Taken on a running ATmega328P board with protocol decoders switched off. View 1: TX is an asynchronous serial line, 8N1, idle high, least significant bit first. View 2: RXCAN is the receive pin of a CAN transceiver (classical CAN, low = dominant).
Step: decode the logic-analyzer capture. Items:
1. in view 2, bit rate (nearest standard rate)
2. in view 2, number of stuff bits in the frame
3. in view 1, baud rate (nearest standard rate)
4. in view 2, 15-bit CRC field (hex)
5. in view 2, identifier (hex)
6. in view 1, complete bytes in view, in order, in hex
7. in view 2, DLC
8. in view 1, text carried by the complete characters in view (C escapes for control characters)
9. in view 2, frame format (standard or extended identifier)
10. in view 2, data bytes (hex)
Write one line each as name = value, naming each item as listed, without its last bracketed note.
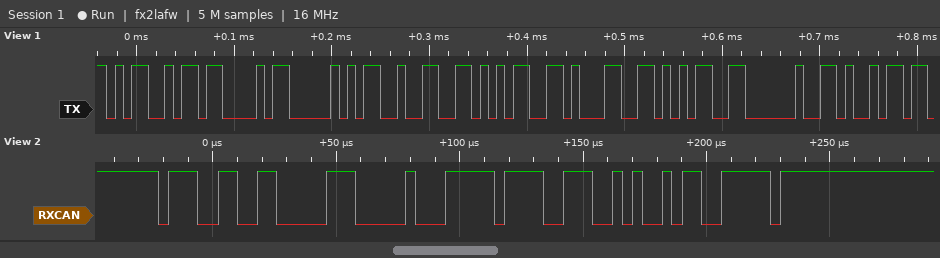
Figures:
in view 2, bit rate = 250 kbit/s
in view 2, number of stuff bits in the frame = 3
in view 1, baud rate = 115200 baud
in view 2, 15-bit CRC field = 0x52CF
in view 2, identifier = 0x733
in view 1, complete bytes in view, in order, in hex = 4D 43 50 32 35 31 35 20 69
in view 2, DLC = 3
in view 1, text carried by the complete characters in view = "MCP2515 i"
in view 2, frame format = standard
in view 2, data bytes = 00 FF 9C
